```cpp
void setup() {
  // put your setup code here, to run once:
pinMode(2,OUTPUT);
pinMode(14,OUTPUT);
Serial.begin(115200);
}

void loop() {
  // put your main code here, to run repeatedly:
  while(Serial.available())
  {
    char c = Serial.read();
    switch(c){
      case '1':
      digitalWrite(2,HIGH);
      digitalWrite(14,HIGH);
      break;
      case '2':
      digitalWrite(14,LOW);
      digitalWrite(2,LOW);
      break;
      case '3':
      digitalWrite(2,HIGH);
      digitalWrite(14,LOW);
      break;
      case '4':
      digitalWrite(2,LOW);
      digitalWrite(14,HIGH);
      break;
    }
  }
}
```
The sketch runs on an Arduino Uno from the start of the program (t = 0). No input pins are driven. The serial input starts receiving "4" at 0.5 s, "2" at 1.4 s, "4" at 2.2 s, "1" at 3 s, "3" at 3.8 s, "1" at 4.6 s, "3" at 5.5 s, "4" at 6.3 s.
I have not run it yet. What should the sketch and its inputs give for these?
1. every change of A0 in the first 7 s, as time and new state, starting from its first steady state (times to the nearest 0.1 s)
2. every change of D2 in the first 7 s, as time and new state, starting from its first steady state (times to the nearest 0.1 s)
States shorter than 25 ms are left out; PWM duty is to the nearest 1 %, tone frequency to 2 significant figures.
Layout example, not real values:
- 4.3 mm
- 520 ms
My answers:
- 0 s low; 0.5 s high; 1.4 s low; 2.2 s high; 3.8 s low; 4.6 s high; 5.5 s low; 6.3 s high
- 0 s low; 3 s high; 6.3 s low
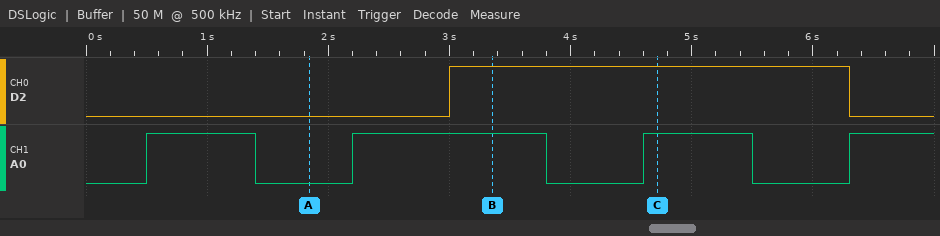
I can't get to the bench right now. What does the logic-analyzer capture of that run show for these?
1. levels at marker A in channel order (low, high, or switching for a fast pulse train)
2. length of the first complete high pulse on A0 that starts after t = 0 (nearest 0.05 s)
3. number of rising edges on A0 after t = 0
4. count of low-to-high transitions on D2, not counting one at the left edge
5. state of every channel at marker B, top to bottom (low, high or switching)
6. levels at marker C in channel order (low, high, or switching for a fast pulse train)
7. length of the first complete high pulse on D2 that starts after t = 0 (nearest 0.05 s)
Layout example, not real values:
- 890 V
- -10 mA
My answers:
- D2 low, A0 low
- 0.90 s
- 4
- 1
- D2 high, A0 high
- D2 high, A0 high
- 3.30 s
